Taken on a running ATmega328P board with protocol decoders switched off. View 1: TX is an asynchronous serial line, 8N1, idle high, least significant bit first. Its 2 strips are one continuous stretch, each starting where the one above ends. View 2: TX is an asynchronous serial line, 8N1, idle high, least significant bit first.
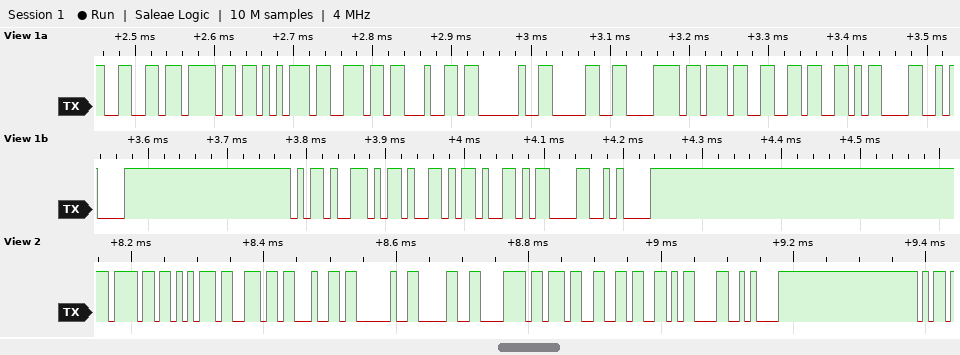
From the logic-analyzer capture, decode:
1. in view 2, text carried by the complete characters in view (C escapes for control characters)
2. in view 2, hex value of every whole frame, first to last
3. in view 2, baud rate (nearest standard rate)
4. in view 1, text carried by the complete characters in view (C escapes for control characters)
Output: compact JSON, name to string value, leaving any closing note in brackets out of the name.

{"in view 2, text carried by the complete characters in view": "\"ound 0x76\\r\\n\"", "in view 2, hex value of every whole frame, first to last": "6F 75 6E 64 20 30 78 37 36 0D 0A", "in view 2, baud rate": "115200 baud", "in view 1, text carried by the complete characters in view": "\"found 0x76\\r\\n---\\r\\n\""}
